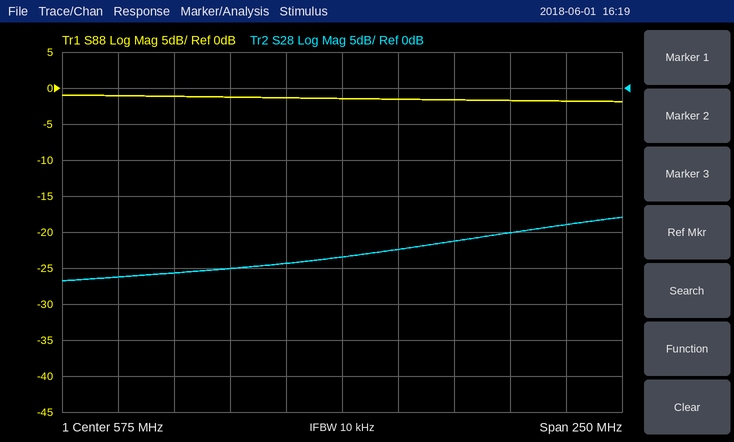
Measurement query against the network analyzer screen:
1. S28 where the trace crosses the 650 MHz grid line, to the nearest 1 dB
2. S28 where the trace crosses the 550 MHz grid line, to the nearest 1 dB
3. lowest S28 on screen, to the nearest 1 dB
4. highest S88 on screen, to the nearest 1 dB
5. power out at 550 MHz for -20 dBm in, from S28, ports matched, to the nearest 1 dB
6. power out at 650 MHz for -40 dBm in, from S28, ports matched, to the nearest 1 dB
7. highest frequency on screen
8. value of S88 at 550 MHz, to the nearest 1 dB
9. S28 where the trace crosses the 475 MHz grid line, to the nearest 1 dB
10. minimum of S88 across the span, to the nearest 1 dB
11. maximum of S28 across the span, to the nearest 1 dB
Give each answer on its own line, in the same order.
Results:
-20 dB
-24 dB
-27 dB
-1 dB
-44 dBm
-60 dBm
700 MHz
-1 dB
-26 dB
-2 dB
-18 dB
